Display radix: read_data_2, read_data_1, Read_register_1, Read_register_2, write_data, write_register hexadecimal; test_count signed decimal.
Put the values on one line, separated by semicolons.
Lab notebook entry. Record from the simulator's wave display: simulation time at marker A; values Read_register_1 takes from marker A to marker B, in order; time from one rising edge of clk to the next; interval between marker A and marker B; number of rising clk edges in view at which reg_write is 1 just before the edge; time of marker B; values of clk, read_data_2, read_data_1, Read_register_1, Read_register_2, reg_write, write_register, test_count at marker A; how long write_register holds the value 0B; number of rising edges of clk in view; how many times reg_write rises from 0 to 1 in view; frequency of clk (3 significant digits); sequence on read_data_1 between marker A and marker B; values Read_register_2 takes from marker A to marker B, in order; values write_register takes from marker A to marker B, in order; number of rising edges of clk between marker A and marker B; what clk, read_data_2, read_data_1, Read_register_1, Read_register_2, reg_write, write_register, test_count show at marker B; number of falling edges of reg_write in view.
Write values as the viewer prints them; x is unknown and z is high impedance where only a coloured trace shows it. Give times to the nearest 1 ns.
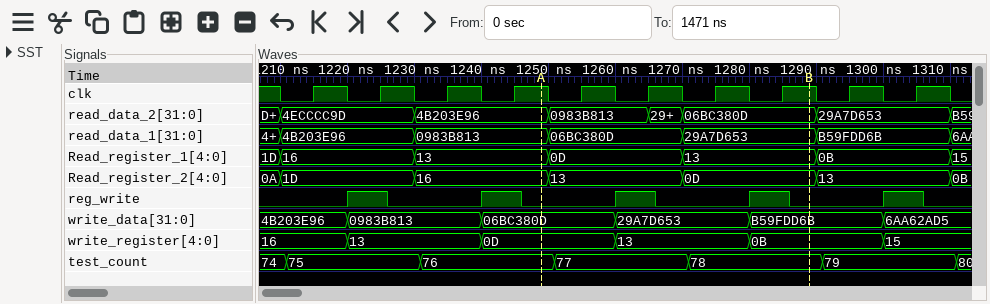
1249 ns; 13, 0D, 13; 10 ns; 40 ns; 5; 1289 ns; clk=1, read_data_2=4B203E96, read_data_1=0983B813, Read_register_1=13, Read_register_2=16, reg_write=0, write_register=0D, test_count=76; 20 ns; 10; 5; 100 MHz; 0983B813, 06BC380D, 29A7D653; 16, 13, 0D; 0D, 13, 0B; 4; clk=1, read_data_2=06BC380D, read_data_1=29A7D653, Read_register_1=13, Read_register_2=0D, reg_write=0, write_register=0B, test_count=78; 5
